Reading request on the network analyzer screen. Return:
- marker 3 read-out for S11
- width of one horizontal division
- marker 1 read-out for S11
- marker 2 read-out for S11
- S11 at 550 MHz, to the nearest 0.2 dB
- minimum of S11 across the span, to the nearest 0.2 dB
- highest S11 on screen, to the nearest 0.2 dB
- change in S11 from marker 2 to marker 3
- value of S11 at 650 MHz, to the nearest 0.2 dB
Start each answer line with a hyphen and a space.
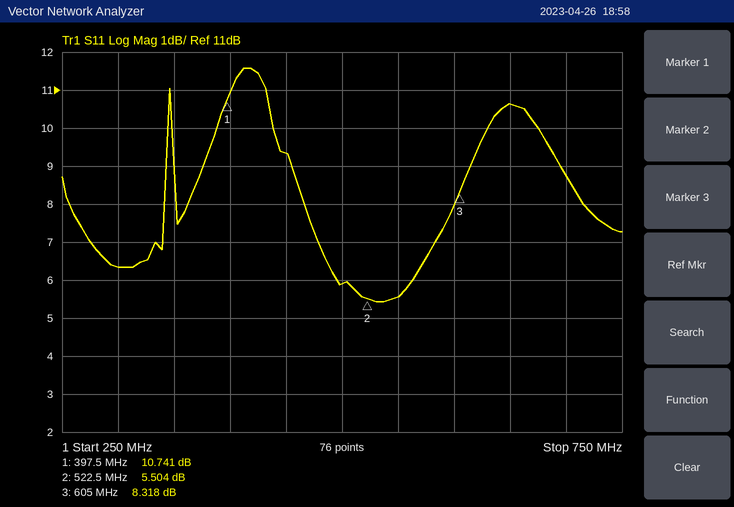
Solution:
- 8.318 dB
- 50 MHz
- 10.741 dB
- 5.504 dB
- 5.6 dB
- 5.4 dB
- 11.6 dB
- 2.814 dB
- 10.6 dB
